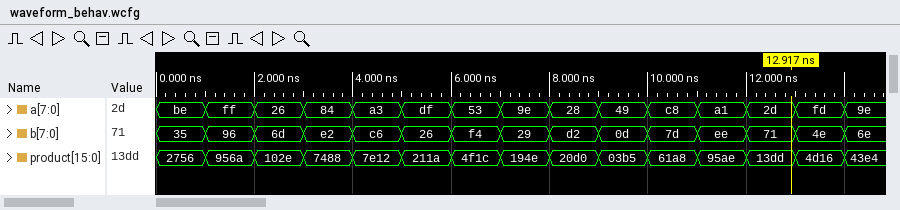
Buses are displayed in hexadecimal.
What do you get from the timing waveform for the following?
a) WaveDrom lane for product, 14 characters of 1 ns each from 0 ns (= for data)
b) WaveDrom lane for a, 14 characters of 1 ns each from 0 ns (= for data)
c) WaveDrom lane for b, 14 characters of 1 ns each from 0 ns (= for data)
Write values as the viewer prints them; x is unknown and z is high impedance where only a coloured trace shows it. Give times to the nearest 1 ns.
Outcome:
{name: 'product', wave: '==============', data: '2756 956a 102e 7488 7e12 211a 4f1c 194e 20d0 03b5 61a8 95ae 13dd 4d16'}
{name: 'a', wave: '==============', data: 'be ff 26 84 a3 df 53 9e 28 49 c8 a1 2d fd'}
{name: 'b', wave: '==============', data: '35 96 6d e2 c6 26 f4 29 d2 0d 7d ee 71 4e'}
